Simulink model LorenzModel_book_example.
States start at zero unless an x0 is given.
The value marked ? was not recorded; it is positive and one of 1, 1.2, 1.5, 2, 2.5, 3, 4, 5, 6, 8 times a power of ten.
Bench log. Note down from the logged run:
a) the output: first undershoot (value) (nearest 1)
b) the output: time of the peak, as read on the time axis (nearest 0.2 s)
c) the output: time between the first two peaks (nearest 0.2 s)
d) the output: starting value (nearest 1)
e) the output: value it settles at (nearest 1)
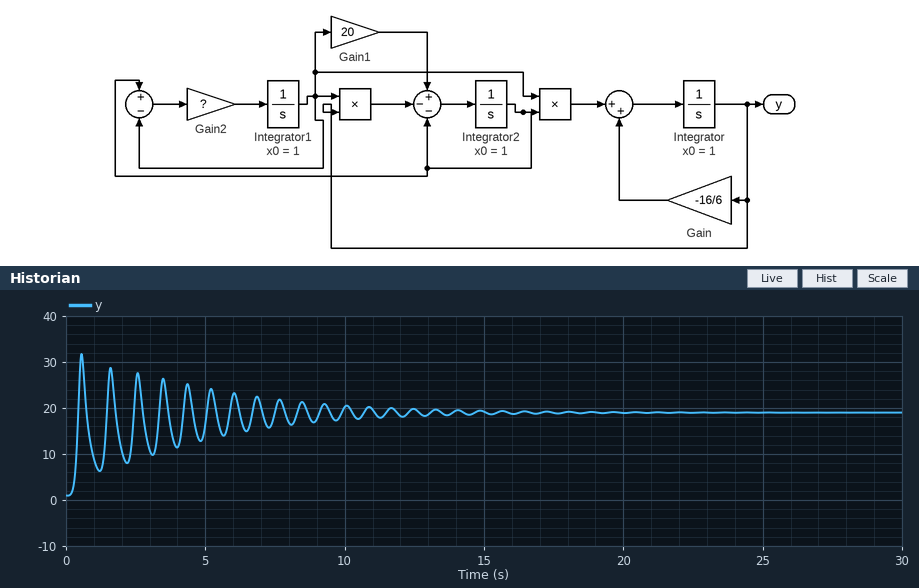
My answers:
6
0.6 s
1.0 s
1
19
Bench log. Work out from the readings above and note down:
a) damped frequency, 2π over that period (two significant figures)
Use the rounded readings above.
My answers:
6.3 rad/s
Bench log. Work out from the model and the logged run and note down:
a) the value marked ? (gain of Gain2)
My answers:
5
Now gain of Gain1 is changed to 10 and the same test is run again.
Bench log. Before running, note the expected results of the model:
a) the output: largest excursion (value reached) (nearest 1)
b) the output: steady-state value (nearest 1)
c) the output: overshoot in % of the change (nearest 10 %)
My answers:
14
9
60 %
